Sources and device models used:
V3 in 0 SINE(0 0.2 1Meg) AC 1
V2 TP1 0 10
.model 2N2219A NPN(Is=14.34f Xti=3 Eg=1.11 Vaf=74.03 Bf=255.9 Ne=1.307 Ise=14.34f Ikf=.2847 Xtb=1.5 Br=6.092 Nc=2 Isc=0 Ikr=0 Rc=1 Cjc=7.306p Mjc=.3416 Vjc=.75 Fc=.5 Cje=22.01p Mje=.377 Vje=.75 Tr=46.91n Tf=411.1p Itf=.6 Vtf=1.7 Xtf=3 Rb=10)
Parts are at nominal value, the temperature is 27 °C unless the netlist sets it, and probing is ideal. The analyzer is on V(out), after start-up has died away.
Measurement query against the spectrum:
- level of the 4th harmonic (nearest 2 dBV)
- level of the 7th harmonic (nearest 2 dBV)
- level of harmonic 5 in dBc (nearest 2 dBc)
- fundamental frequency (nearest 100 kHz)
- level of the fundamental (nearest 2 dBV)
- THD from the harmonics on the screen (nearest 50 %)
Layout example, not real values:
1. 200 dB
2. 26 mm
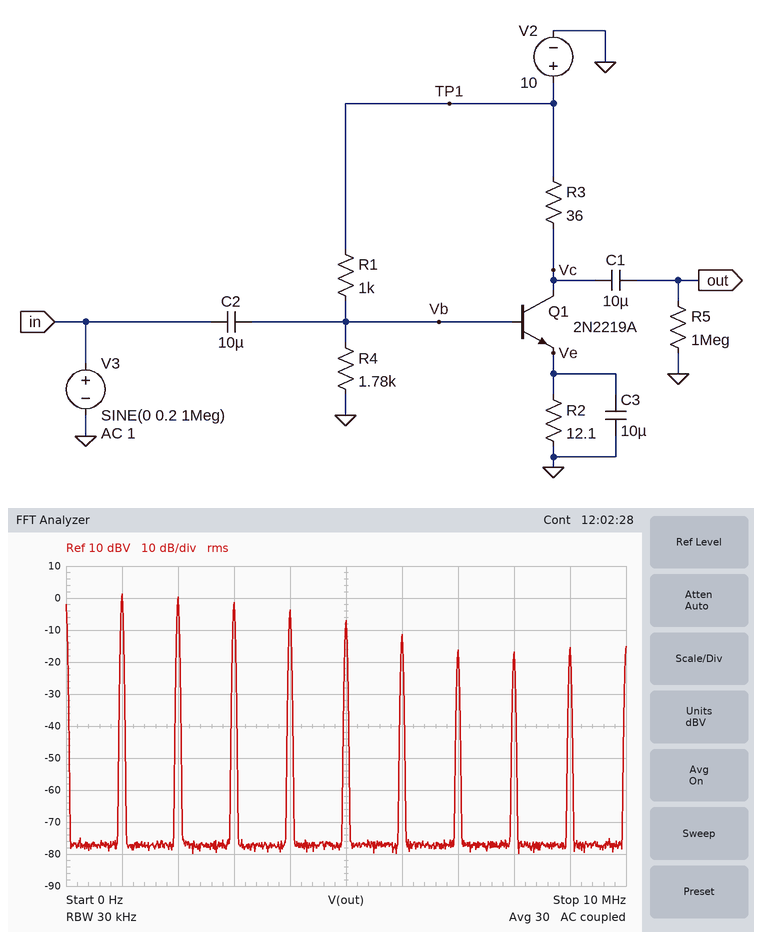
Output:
1. -4 dBV
2. -16 dBV
3. -8 dBc
4. 1.0 MHz
5. 2 dBV
6. 150 %
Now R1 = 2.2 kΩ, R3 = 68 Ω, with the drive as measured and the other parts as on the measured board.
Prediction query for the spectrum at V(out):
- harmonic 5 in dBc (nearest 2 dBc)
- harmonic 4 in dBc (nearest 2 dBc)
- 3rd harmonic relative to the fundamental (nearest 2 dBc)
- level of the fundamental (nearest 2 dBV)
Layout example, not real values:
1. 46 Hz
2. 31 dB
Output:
1. -24 dBc
2. -12 dBc
3. -6 dBc
4. 6 dBV
